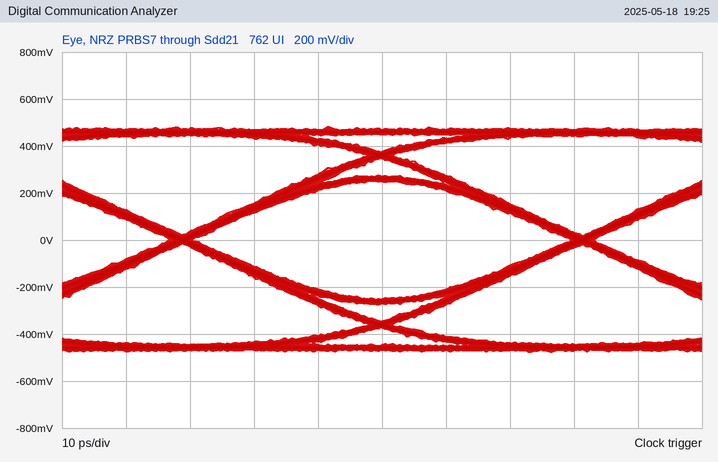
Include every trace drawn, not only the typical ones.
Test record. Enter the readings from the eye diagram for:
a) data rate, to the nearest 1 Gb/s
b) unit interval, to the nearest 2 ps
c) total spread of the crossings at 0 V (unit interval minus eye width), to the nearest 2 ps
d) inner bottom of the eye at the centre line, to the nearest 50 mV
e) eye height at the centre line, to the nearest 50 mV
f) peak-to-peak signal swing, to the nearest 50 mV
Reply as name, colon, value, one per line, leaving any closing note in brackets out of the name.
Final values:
data rate, to the nearest 1 Gb/s: 16 Gb/s
unit interval, to the nearest 2 ps: 62 ps
total spread of the crossings at 0 V (unit interval minus eye width), to the nearest 2 ps: 4 ps
inner bottom of the eye at the centre line, to the nearest 50 mV: -250 mV
eye height at the centre line, to the nearest 50 mV: 500 mV
peak-to-peak signal swing, to the nearest 50 mV: 950 mV
